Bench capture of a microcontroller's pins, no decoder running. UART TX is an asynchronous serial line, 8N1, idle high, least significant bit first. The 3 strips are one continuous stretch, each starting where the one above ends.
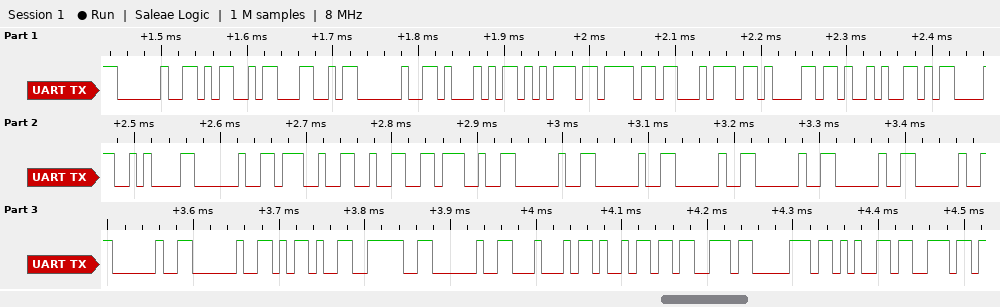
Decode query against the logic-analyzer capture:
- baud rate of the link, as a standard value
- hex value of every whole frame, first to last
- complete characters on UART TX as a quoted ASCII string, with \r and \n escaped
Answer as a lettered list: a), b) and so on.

a) 115200 baud
b) 0x20 0x4D 0x4C 0x20 0x51 0x75 0x6F 0x74 0x61 0x29 0x0D 0x0A 0x20 0x27 0x32 0x27 0x20 0x20 0x20 0x20 0x20 0x20 0x20 0x20 0x2D 0x3E 0x20 0x44 0x69 0x73 0x70 0x65 0x6E
c) " ML Quota)\r\n '2'        -> Dispen"
